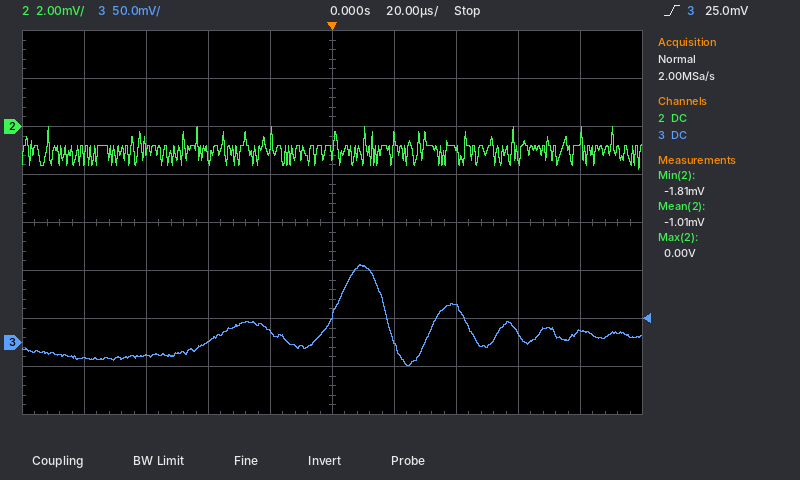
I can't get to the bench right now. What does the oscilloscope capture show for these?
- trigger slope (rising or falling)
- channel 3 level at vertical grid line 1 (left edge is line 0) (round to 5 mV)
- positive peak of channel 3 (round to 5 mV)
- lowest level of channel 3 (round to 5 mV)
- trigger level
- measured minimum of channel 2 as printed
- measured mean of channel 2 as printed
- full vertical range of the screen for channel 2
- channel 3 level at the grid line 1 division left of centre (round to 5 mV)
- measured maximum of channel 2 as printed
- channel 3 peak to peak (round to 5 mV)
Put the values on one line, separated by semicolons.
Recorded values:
rising; -15 mV; 80 mV; -25 mV; 25.0 mV; -1.81 mV; -1.01 mV; 16 mV; 10 mV; 0.00 V; 105 mV
